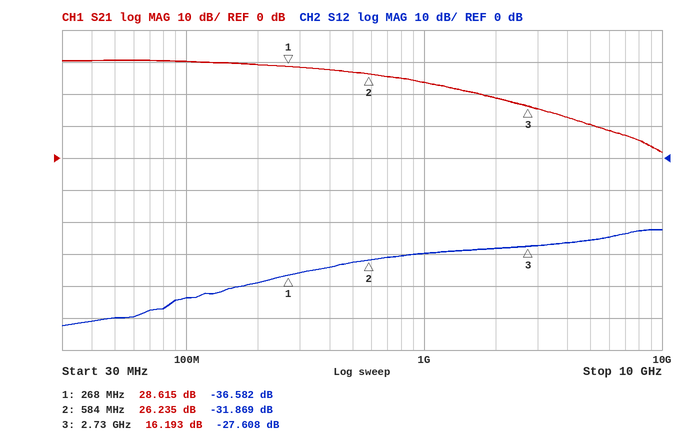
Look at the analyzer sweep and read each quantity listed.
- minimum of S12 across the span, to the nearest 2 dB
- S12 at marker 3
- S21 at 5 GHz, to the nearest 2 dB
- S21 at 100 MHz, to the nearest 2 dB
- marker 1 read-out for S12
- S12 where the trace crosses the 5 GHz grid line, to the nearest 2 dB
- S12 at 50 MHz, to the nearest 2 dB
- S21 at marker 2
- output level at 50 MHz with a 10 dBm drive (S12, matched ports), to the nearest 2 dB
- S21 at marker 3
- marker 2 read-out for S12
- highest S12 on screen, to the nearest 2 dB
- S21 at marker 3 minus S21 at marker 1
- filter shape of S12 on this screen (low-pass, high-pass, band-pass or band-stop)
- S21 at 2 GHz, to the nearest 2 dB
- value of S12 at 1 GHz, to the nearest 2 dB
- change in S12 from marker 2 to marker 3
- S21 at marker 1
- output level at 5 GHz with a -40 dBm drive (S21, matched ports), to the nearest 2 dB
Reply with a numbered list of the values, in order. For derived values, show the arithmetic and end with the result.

1. -52 dB
2. -27.608 dB
3. 10 dB
4. 30 dB
5. -36.582 dB
6. -26 dB
7. -50 dB
8. 26.235 dB
9. 10 dBm + (-50 dB) = -40 dBm
10. 16.193 dB
11. -31.869 dB
12. -22 dB
13. 16.193 − (28.615) = -12.422 dB
14. high-pass
15. 18 dB
16. -30 dB
17. -27.608 − (-31.869) = 4.261 dB
18. 28.615 dB
19. -40 dBm + (10 dB) = -30 dBm
